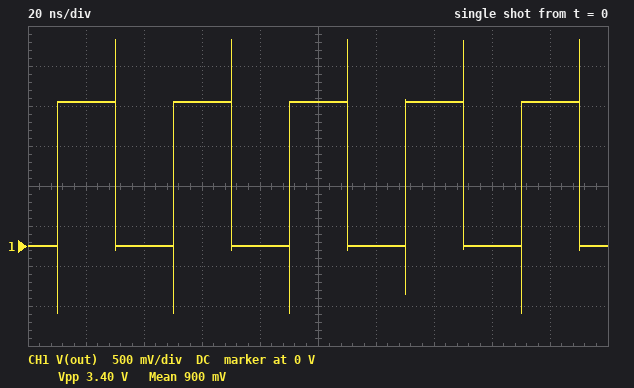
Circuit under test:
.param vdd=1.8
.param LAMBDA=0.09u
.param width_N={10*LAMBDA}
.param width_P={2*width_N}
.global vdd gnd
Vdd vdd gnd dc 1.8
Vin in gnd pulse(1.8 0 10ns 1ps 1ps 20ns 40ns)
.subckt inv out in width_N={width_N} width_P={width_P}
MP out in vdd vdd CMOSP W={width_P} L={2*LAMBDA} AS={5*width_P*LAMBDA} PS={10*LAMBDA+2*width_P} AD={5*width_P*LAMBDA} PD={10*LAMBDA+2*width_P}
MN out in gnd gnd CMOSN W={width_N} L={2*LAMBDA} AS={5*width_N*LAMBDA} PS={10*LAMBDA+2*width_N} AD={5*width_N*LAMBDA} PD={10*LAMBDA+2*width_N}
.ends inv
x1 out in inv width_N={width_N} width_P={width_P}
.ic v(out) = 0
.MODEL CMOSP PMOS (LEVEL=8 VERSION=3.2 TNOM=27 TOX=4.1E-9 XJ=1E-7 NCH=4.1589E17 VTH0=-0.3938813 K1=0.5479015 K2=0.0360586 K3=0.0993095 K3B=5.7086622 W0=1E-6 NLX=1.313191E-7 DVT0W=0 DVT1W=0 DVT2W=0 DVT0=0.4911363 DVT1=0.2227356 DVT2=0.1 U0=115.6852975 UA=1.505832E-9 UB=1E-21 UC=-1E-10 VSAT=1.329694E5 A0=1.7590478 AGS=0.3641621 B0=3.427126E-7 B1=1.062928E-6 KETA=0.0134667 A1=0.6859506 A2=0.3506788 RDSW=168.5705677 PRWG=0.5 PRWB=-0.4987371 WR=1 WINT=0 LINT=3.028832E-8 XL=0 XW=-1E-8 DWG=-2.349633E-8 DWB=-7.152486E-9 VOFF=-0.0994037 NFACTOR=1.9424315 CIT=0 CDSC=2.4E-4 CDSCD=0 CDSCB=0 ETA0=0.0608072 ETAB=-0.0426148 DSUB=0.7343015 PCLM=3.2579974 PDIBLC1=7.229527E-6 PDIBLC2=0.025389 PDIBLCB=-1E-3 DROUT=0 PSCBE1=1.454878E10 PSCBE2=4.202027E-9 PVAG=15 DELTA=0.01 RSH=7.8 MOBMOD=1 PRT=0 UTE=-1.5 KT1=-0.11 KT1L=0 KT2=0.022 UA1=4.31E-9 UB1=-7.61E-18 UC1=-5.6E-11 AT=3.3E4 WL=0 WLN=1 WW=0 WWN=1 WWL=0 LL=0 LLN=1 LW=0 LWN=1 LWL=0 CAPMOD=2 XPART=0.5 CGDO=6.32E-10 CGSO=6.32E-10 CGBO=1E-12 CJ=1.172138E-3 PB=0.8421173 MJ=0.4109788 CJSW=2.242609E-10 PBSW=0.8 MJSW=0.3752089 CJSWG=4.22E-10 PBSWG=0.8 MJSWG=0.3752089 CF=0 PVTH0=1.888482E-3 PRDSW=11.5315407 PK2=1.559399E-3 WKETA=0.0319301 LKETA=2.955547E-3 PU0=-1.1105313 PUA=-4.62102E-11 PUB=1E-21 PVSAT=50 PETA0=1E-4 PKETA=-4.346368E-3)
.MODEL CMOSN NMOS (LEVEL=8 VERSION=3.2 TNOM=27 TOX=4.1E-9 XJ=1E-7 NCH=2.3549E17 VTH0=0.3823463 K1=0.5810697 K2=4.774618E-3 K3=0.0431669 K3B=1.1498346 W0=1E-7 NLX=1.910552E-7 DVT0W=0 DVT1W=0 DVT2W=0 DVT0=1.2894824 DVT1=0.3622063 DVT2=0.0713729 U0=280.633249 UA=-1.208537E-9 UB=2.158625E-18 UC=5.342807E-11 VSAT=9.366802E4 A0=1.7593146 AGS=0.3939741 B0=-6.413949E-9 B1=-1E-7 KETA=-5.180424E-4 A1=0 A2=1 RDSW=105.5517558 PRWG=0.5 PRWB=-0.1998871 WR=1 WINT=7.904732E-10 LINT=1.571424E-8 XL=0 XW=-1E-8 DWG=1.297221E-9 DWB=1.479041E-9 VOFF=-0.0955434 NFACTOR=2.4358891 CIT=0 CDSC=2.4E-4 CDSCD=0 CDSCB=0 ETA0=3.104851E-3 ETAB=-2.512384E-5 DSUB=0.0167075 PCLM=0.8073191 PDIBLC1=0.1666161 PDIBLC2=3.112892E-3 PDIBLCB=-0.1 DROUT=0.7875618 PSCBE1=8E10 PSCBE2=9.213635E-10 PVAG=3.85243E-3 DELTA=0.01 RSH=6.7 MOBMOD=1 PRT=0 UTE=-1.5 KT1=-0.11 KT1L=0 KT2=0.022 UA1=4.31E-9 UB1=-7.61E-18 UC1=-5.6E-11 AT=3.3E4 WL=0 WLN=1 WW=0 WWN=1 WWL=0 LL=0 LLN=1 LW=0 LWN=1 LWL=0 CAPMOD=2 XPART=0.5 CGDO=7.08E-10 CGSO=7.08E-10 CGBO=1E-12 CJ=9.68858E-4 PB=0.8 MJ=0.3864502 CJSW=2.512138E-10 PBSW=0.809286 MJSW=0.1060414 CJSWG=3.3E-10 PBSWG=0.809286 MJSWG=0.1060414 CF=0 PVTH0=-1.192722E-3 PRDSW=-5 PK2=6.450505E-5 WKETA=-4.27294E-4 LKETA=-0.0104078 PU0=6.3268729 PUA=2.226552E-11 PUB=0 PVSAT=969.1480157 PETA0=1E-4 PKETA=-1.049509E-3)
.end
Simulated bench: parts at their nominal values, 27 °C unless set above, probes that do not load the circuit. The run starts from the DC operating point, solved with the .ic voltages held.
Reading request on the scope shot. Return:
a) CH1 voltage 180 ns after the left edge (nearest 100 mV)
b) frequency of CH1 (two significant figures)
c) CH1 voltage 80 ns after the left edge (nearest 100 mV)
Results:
1.8 V
25 MHz
0 V
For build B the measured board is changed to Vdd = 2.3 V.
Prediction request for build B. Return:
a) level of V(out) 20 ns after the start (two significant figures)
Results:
2.3 V
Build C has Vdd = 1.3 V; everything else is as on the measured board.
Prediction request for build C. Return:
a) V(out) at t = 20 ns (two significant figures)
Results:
1.3 V
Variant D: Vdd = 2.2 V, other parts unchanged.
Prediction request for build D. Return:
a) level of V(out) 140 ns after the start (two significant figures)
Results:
2.2 V
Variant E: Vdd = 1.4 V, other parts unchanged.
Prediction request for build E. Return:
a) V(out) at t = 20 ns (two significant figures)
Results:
1.4 V
